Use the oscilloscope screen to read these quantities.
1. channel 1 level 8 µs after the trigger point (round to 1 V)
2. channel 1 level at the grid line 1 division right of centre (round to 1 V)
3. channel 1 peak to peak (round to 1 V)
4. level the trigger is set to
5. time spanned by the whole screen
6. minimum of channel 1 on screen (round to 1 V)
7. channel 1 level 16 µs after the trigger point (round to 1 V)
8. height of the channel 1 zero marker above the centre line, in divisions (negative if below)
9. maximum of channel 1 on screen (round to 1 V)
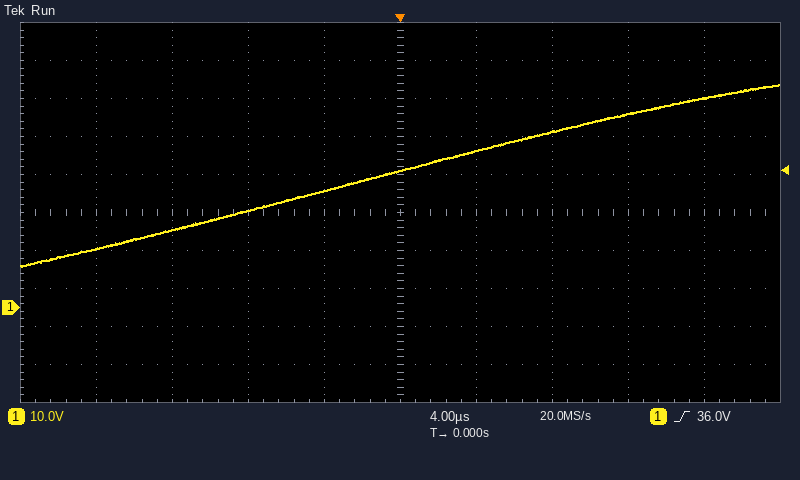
46 V
41 V
48 V
36.0 V
40 µs
11 V
55 V
-2.5 div
59 V
